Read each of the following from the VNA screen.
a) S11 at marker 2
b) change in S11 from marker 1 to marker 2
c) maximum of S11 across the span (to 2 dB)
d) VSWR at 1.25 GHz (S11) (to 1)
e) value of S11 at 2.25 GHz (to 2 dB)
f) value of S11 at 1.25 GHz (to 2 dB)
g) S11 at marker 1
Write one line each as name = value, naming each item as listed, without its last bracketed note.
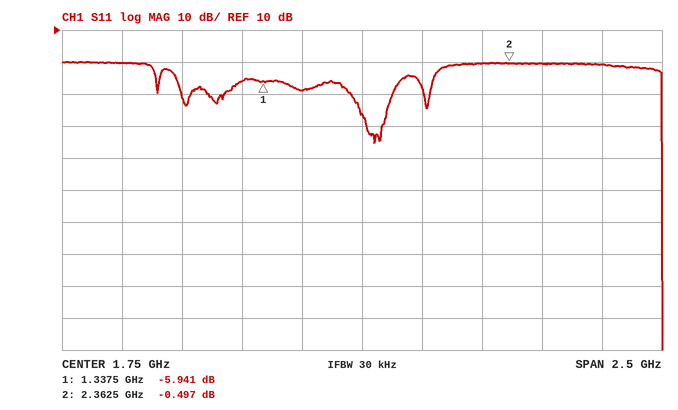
S11 at marker 2 = -0.497 dB
change in S11 from marker 1 to marker 2 = 5.444 dB
maximum of S11 across the span = 0 dB
VSWR at 1.25 GHz (S11) = 3
value of S11 at 2.25 GHz = 0 dB
value of S11 at 1.25 GHz = -6 dB
S11 at marker 1 = -5.941 dB
